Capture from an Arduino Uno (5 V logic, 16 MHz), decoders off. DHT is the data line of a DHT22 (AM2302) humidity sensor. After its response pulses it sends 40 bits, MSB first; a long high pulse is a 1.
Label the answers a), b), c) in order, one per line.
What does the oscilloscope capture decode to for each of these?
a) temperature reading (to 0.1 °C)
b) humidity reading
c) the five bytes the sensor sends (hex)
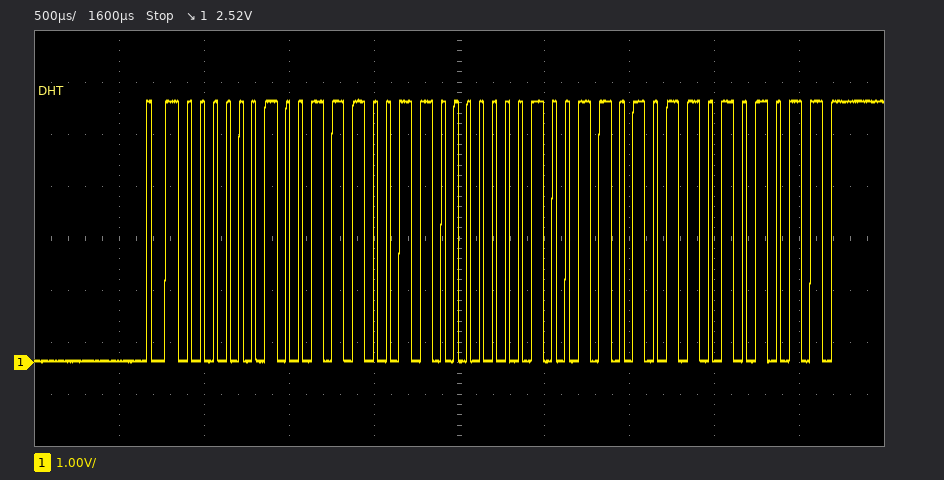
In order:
a) 30.9 °C
b) 62.7 %
c) 02 73 01 35 AB
